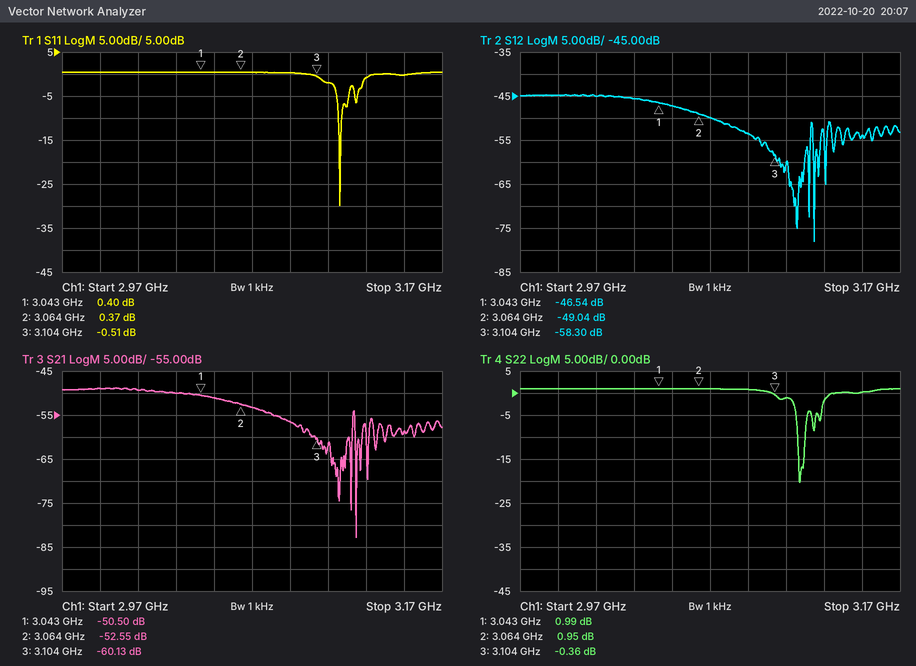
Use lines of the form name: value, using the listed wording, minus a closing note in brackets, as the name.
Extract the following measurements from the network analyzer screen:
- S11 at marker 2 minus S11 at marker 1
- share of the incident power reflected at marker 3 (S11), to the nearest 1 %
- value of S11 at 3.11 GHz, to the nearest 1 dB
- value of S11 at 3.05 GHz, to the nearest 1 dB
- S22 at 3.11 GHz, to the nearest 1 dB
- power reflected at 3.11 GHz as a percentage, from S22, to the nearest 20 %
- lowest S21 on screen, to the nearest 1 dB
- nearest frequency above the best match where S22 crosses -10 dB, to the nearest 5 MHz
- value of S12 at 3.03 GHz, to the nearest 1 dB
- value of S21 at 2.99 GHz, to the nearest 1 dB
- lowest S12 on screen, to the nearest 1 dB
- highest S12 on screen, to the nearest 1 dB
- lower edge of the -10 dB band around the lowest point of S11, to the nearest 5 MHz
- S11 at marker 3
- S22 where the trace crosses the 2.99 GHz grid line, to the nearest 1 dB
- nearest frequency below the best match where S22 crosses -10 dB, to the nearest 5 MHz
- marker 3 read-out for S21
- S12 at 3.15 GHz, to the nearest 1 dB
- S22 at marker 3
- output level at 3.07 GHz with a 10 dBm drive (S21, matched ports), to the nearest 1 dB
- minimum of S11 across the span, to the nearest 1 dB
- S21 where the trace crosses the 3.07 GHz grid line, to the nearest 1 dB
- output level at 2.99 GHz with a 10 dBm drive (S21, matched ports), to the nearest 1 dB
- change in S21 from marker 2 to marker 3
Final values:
S11 at marker 2 minus S11 at marker 1: -0.03 dB
share of the incident power reflected at marker 3 (S11), to the nearest 1 %: 89 %
value of S11 at 3.11 GHz, to the nearest 1 dB: -2 dB
value of S11 at 3.05 GHz, to the nearest 1 dB: 0 dB
S22 at 3.11 GHz, to the nearest 1 dB: -1 dB
power reflected at 3.11 GHz as a percentage, from S22, to the nearest 20 %: 80 %
lowest S21 on screen, to the nearest 1 dB: -83 dB
nearest frequency above the best match where S22 crosses -10 dB, to the nearest 5 MHz: 3.120 GHz
value of S12 at 3.03 GHz, to the nearest 1 dB: -46 dB
value of S21 at 2.99 GHz, to the nearest 1 dB: -49 dB
lowest S12 on screen, to the nearest 1 dB: -78 dB
highest S12 on screen, to the nearest 1 dB: -45 dB
lower edge of the -10 dB band around the lowest point of S11, to the nearest 5 MHz: 3.115 GHz
S11 at marker 3: -0.51 dB
S22 where the trace crosses the 2.99 GHz grid line, to the nearest 1 dB: 1 dB
nearest frequency below the best match where S22 crosses -10 dB, to the nearest 5 MHz: 3.115 GHz
marker 3 read-out for S21: -60.13 dB
S12 at 3.15 GHz, to the nearest 1 dB: -54 dB
S22 at marker 3: -0.36 dB
output level at 3.07 GHz with a 10 dBm drive (S21, matched ports), to the nearest 1 dB: -43 dBm
minimum of S11 across the span, to the nearest 1 dB: -30 dB
S21 where the trace crosses the 3.07 GHz grid line, to the nearest 1 dB: -53 dB
output level at 2.99 GHz with a 10 dBm drive (S21, matched ports), to the nearest 1 dB: -39 dBm
change in S21 from marker 2 to marker 3: -7.58 dB
